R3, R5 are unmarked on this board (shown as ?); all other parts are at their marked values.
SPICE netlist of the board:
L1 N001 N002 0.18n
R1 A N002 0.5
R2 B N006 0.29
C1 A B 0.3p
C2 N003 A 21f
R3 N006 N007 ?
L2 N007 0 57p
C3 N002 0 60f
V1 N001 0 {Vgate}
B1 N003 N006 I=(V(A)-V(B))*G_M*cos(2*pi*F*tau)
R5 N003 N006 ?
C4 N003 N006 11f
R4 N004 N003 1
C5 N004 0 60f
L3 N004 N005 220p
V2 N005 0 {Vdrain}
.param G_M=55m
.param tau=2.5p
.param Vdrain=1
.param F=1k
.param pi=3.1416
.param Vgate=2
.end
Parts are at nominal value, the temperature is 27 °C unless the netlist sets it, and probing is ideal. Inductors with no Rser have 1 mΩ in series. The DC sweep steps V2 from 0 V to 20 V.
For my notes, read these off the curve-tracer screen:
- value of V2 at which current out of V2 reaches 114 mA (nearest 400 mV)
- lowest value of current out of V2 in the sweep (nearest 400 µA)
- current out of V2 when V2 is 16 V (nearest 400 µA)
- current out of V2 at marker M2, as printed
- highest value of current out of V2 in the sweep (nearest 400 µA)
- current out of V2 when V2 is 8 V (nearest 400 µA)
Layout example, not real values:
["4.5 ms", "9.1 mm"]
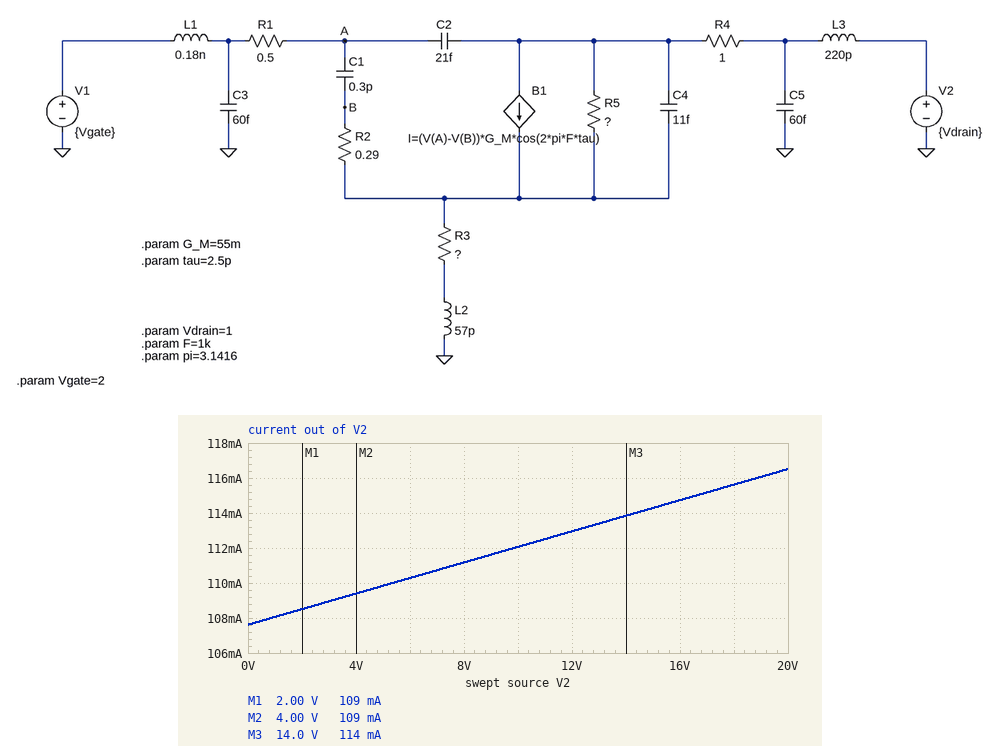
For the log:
["14.4 V", "107.6 mA", "114.8 mA", "109 mA", "116.4 mA", "111.2 mA"]
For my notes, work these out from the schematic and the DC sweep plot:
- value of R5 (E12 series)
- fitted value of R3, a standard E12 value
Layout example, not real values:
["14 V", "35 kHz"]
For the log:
["2.2 kΩ", "0.39 Ω"]
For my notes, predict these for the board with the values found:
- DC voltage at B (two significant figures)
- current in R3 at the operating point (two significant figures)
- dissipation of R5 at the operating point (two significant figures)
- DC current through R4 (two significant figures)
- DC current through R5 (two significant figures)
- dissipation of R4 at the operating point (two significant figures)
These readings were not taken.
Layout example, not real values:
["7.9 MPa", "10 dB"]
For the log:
["42 mV", "110 mA", "330 µW", "110 mA", "390 µA", "12 mW"]
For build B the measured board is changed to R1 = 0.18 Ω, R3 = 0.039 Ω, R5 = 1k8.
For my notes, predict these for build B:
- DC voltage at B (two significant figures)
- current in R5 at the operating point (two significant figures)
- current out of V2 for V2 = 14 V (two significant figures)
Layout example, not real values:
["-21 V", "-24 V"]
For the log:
["4.4 mV", "490 µA", "120 mA"]
